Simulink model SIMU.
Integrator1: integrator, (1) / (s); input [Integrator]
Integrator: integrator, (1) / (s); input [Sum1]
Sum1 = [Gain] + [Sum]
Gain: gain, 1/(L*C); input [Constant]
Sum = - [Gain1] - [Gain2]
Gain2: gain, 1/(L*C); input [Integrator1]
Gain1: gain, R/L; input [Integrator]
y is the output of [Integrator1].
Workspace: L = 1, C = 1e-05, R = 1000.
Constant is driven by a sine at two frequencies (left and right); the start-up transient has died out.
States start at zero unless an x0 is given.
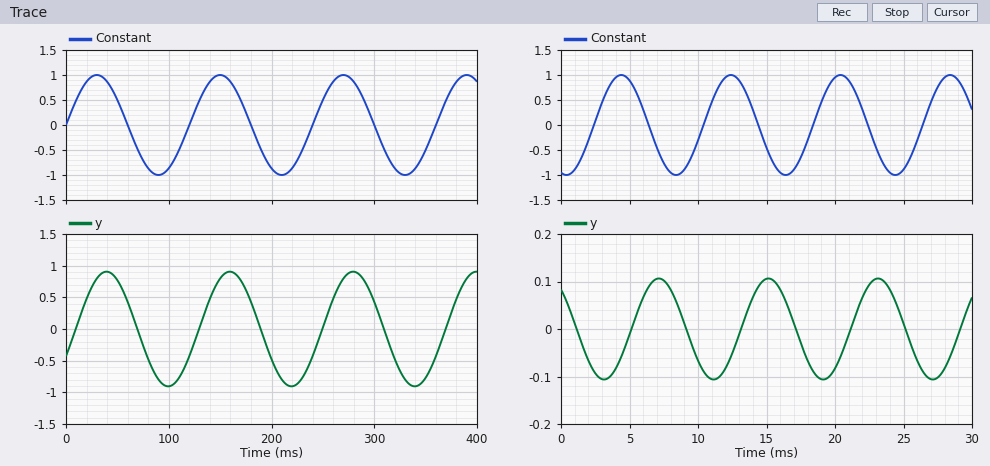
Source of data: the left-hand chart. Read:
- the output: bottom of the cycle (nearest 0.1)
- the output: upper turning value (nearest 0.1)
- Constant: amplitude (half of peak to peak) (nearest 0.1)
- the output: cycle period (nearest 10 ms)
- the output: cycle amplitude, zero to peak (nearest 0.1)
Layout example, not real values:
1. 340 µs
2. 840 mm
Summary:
1. -0.9
2. 0.9
3. 1.0
4. 120 ms
5. 0.9
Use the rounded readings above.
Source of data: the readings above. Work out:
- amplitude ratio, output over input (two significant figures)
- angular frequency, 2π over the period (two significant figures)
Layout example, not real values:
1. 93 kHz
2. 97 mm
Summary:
1. 0.90
2. 0.052 rad/ms
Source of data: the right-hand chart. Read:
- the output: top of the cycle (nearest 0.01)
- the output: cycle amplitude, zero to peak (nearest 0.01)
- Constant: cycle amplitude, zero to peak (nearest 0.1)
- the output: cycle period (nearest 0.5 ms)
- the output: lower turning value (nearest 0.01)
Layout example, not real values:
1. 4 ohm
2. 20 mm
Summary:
1. 0.11
2. 0.11
3. 1.0
4. 8.0 ms
5. -0.11
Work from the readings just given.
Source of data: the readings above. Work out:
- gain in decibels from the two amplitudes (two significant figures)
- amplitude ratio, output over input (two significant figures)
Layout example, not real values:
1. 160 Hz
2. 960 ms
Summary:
1. -19 dB
2. 0.11
